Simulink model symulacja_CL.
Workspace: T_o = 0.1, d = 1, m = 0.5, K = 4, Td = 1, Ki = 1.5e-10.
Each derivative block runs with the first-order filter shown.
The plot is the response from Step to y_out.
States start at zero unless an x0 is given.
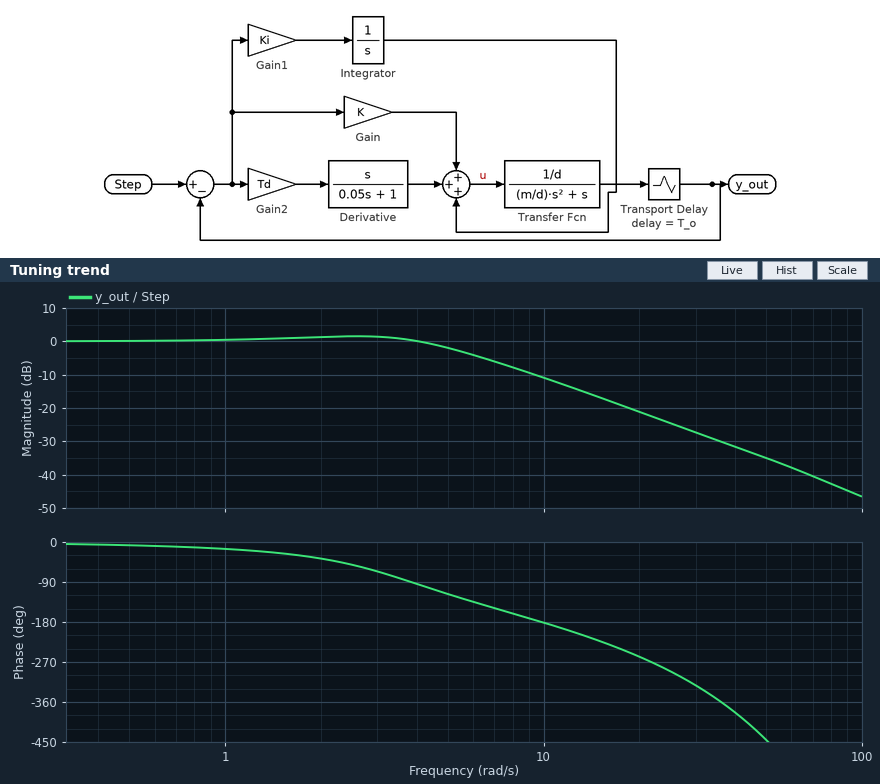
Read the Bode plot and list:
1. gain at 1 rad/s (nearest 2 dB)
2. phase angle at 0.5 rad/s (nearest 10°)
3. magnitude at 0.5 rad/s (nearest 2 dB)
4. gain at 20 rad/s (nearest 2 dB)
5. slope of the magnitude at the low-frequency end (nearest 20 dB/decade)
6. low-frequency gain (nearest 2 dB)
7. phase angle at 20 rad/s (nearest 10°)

0 dB
-10°
0 dB
-22 dB
0 dB/decade
0 dB
-260°
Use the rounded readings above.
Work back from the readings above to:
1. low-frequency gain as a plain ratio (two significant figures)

1.0
